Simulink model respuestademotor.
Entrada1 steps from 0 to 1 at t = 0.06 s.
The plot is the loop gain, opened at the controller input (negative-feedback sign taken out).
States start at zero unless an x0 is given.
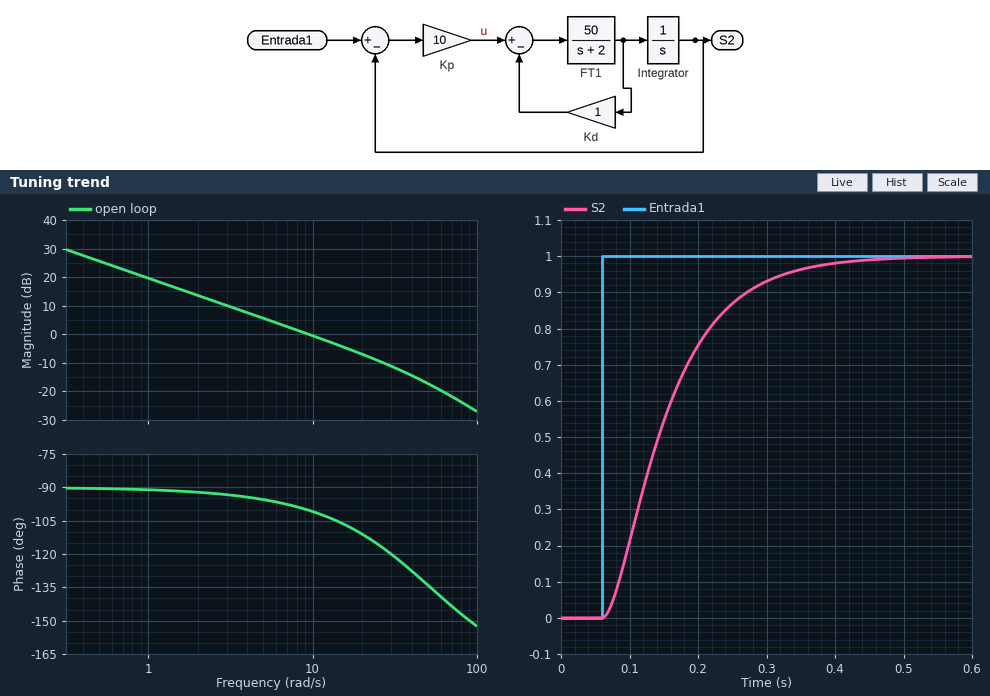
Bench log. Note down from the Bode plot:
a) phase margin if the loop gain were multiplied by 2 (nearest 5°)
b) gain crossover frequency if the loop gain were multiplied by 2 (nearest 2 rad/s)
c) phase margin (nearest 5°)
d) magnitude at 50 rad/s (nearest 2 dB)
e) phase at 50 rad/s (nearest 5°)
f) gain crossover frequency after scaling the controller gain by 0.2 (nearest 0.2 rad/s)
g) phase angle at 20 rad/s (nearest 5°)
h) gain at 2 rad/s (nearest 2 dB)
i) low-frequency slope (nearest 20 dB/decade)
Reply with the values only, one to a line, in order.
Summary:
70°
18 rad/s
80°
-18 dB
-135°
2.0 rad/s
-110°
14 dB
-20 dB/decade
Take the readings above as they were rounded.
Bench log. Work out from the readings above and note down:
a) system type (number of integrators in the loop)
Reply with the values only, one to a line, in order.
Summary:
1
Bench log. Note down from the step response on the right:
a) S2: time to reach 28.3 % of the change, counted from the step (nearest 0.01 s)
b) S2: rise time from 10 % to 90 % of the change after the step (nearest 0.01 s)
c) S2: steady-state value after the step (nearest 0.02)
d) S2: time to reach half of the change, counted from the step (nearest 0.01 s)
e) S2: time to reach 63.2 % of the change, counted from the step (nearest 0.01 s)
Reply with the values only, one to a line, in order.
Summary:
0.05 s
0.19 s
1.00
0.08 s
0.11 s
